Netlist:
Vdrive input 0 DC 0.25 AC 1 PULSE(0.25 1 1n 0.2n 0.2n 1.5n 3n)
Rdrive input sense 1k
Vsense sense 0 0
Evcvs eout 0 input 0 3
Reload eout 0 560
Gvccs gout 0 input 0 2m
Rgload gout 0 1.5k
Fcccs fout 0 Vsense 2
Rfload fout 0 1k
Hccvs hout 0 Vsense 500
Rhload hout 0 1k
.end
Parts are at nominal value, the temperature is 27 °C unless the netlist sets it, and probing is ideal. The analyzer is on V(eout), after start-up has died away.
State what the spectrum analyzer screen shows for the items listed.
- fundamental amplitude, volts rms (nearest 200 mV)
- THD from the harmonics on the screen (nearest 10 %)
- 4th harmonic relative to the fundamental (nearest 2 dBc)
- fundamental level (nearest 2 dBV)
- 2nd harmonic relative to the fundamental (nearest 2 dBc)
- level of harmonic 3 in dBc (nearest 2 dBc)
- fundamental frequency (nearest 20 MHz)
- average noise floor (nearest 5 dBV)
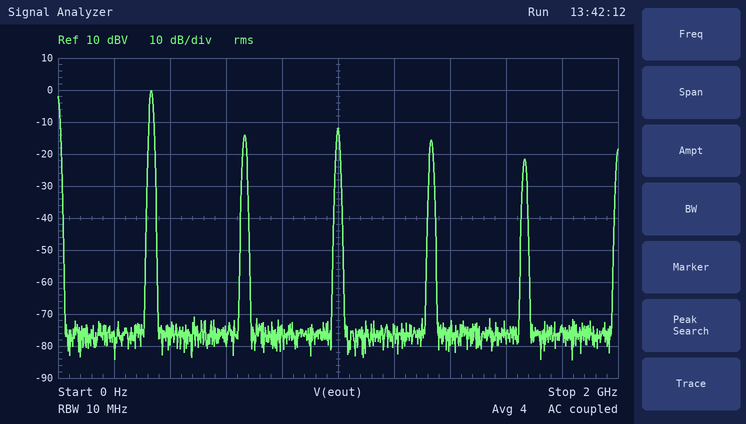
1.0 V
40 %
-16 dBc
0 dBV
-14 dBc
-12 dBc
340 MHz
-75 dBV
